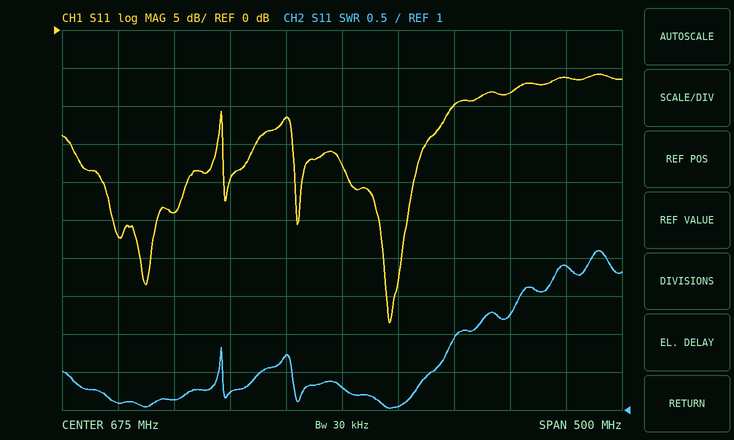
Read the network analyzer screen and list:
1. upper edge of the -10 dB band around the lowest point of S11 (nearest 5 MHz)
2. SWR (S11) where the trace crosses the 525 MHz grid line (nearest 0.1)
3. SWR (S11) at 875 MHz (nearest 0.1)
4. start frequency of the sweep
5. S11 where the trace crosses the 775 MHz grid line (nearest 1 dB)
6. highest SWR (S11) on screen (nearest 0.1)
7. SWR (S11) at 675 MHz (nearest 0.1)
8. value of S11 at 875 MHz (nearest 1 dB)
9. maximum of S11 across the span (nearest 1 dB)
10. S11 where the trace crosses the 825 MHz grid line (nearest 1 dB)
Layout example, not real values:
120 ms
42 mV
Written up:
775 MHz
1.1
2.9
425 MHz
-10 dB
3.1
1.3
-6 dB
-6 dB
-8 dB
